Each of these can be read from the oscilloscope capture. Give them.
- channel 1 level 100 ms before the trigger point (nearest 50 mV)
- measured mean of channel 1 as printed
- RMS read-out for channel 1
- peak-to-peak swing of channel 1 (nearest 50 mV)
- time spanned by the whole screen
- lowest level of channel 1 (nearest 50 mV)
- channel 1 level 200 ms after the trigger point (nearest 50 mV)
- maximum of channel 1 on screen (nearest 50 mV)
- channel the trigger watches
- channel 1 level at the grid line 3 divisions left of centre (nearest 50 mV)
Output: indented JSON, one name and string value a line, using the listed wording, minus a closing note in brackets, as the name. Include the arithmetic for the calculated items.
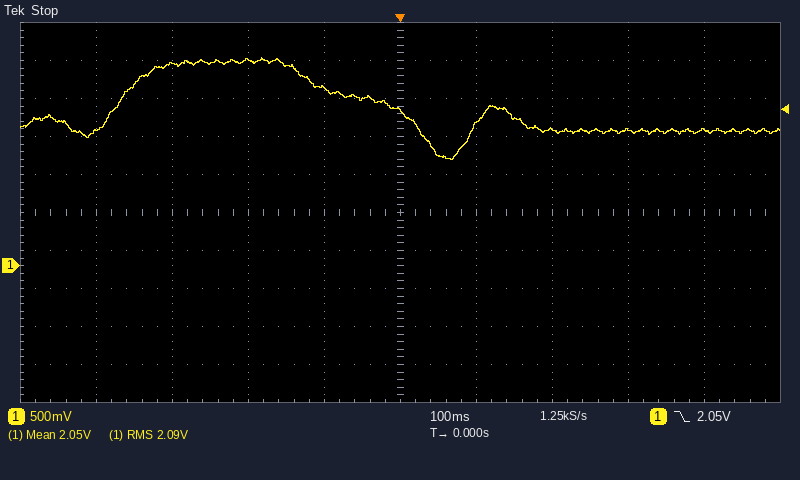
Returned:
{
  "channel 1 level 100 ms before the trigger point": "2.35 V",
  "measured mean of channel 1 as printed": "2.05 V",
  "RMS read-out for channel 1": "2.09 V",
  "peak-to-peak swing of channel 1": "2.75 V − (1.40 V) = 1.35 V",
  "time spanned by the whole screen": "1 s",
  "lowest level of channel 1": "1.40 V",
  "channel 1 level 200 ms after the trigger point": "1.80 V",
  "maximum of channel 1 on screen": "2.75 V",
  "channel the trigger watches": "channel 1",
  "channel 1 level at the grid line 3 divisions left of centre": "2.65 V"
}
